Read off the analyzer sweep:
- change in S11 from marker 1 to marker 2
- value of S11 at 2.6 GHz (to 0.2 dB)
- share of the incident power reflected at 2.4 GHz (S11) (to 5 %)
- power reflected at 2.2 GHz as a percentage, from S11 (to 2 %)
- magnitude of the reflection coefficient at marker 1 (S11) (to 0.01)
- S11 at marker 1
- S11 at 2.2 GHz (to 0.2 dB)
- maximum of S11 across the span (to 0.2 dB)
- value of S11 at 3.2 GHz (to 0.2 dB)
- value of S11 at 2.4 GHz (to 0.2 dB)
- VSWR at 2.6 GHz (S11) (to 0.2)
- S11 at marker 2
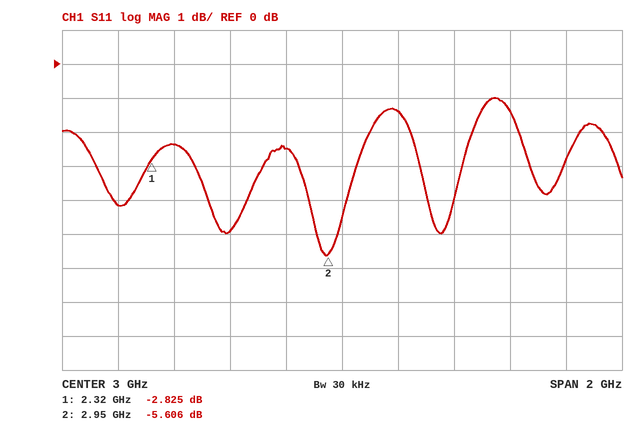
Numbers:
-2.781 dB
-5.0 dB
60 %
38 %
0.72
-2.825 dB
-4.2 dB
-1.0 dB
-1.4 dB
-2.4 dB
3.6
-5.606 dB
